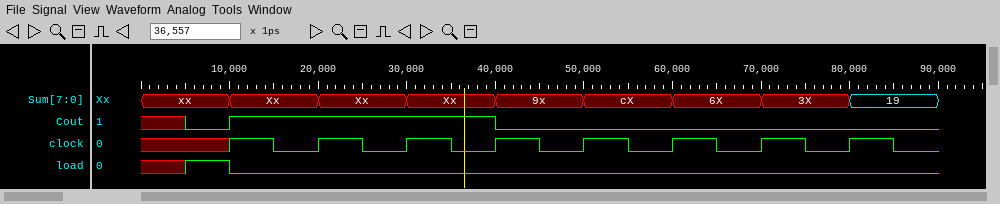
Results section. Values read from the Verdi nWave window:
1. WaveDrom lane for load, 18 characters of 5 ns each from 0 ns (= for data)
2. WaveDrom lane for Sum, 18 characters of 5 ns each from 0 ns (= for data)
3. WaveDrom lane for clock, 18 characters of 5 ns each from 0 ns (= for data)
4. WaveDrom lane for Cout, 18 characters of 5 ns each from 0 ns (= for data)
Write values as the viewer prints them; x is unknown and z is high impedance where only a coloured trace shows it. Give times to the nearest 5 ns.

{name: 'load', wave: 'x10...............'}
{name: 'Sum', wave: 'x.=.=.=.=.=.=.=.=.', data: 'Xx Xx Xx 9x cX 6X 3X 19'}
{name: 'clock', wave: 'x.1010101010101010'}
{name: 'Cout', wave: 'x01.....0.........'}
